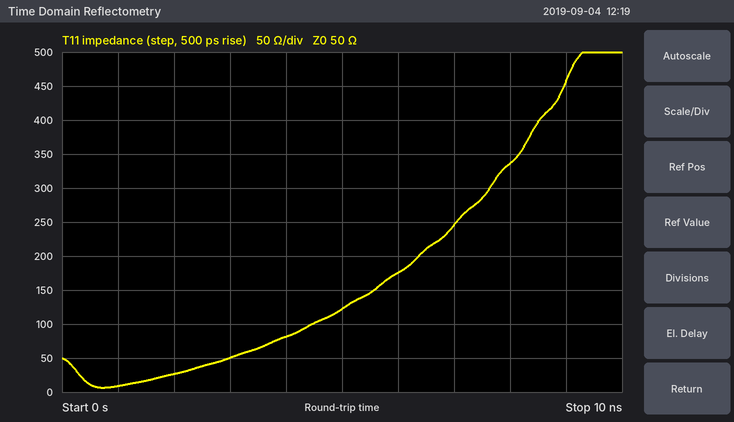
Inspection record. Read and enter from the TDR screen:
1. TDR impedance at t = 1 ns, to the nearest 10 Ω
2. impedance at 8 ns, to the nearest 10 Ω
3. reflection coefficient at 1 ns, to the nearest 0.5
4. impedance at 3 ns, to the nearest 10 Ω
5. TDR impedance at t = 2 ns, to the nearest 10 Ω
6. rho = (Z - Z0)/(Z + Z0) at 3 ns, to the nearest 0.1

10 Ω
340 Ω
-0.5
50 Ω
30 Ω
0.0
